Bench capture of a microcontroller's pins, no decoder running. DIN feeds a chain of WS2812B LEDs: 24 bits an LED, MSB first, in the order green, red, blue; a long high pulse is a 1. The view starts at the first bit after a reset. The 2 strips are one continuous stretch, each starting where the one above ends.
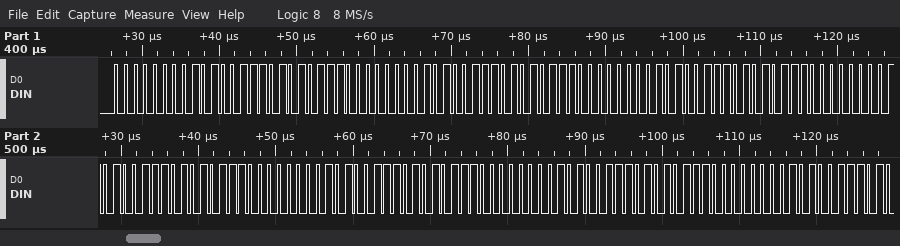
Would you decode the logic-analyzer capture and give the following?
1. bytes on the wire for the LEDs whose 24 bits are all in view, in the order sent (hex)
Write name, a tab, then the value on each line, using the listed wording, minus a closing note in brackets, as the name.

bytes on the wire for the LEDs whose 24 bits are all in view, in the order sent	00 A7 57 00 A7 57 00 A7 57 00 A7 57 00 A7 57 00 A7 57
